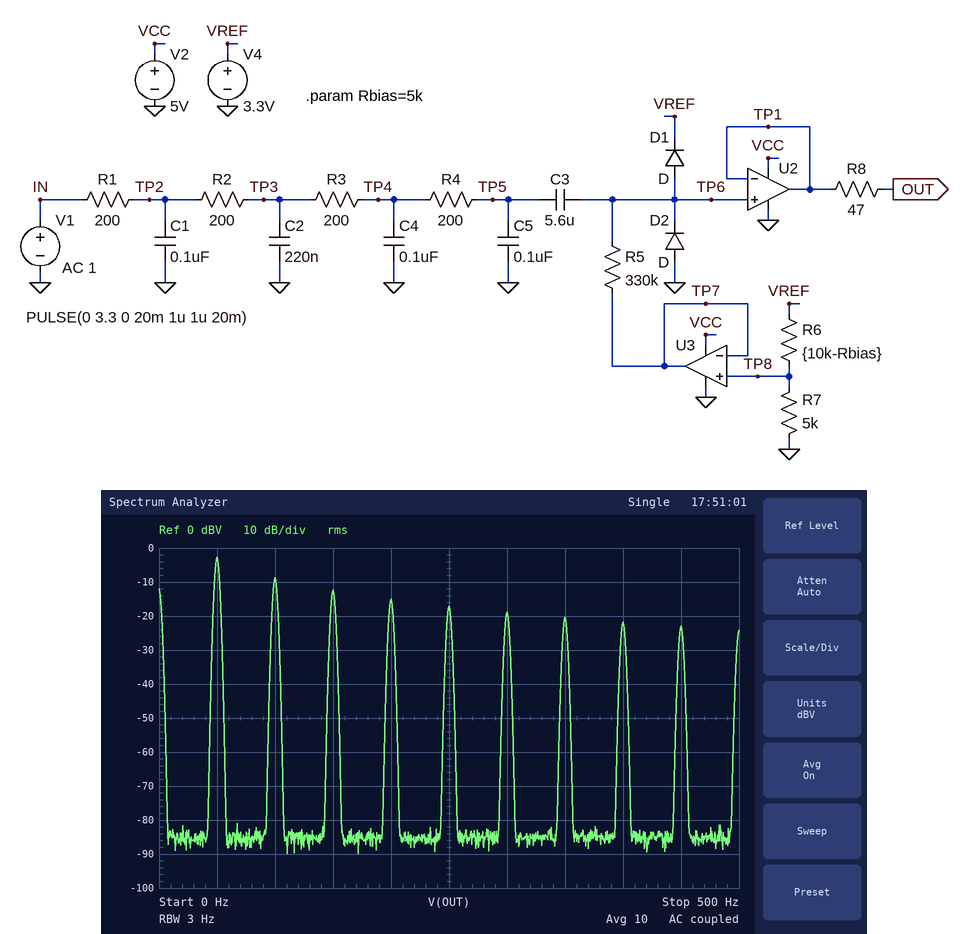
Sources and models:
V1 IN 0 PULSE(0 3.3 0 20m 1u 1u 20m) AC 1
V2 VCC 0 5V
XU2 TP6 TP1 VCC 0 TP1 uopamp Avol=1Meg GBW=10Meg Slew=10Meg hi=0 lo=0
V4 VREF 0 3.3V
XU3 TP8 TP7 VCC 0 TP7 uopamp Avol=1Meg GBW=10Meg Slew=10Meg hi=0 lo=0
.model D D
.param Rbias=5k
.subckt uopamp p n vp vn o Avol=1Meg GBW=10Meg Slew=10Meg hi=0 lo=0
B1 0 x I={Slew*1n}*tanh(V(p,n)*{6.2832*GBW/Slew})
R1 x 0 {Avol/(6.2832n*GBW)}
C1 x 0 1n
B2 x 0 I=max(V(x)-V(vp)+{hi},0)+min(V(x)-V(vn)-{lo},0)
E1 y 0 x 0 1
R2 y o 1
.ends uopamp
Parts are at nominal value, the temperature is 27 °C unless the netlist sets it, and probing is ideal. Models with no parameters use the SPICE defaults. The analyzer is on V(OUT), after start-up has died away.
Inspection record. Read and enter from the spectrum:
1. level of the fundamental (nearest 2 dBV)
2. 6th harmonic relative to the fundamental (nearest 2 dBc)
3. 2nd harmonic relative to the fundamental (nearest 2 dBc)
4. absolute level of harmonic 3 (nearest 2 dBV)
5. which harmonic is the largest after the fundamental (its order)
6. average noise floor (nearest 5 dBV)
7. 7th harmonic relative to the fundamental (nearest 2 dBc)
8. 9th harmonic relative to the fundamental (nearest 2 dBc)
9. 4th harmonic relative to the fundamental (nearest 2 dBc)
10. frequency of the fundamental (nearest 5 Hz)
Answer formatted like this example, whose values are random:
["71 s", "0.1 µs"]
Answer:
["-2 dBV", "-16 dBc", "-6 dBc", "-12 dBV", "2", "-85 dBV", "-18 dBc", "-20 dBc", "-12 dBc", "50 Hz"]
